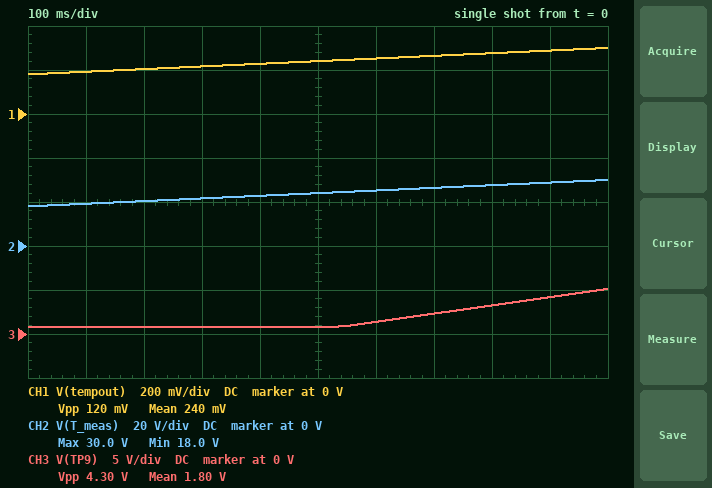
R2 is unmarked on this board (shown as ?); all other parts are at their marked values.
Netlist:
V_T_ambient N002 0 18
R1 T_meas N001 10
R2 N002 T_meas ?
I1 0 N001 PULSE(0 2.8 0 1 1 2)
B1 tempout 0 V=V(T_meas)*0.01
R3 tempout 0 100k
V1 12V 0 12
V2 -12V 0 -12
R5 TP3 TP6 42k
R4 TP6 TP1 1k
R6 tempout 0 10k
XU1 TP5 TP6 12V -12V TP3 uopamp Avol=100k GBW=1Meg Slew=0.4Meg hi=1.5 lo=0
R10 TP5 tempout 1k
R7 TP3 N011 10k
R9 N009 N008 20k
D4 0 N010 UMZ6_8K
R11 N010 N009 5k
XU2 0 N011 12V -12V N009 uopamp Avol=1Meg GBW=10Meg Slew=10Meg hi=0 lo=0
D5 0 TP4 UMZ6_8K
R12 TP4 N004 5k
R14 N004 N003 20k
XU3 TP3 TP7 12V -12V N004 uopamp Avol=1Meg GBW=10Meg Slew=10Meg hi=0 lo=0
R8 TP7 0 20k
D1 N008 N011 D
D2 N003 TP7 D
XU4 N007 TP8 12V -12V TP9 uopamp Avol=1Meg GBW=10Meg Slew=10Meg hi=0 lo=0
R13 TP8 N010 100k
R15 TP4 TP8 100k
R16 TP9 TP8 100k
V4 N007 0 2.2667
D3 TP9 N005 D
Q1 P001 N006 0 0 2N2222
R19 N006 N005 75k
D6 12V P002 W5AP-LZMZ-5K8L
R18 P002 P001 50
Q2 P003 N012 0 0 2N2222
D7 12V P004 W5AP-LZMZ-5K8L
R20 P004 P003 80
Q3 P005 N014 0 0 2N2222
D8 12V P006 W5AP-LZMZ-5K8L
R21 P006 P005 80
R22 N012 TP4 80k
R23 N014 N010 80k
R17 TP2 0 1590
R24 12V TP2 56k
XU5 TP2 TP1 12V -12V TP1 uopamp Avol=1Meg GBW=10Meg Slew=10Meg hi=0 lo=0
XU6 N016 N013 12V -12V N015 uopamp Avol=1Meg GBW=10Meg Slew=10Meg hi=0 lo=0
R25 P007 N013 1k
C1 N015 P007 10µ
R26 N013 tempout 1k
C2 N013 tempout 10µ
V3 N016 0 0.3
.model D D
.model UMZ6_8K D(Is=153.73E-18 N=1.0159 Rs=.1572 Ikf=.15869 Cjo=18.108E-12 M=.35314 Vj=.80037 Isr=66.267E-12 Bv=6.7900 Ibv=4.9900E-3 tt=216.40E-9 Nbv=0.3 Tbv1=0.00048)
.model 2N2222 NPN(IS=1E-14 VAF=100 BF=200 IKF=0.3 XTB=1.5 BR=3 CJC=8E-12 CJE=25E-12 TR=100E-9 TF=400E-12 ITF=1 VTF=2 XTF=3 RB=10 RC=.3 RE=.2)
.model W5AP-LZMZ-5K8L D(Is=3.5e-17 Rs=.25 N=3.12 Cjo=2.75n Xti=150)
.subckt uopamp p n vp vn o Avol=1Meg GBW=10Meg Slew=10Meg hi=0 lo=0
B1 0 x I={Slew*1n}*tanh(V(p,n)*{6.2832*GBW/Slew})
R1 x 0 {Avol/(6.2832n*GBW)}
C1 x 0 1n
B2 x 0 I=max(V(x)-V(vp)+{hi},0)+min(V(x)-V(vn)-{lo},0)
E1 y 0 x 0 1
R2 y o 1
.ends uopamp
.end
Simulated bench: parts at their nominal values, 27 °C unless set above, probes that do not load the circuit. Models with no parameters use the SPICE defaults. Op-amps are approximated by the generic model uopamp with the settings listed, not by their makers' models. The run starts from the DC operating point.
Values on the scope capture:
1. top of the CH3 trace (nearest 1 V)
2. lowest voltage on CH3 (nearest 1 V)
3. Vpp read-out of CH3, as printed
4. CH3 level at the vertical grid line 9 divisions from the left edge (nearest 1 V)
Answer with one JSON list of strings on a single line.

["5 V", "1 V", "4.30 V", "4 V"]
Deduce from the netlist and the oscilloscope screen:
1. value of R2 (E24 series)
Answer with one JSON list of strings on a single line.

["4.3 Ω"]
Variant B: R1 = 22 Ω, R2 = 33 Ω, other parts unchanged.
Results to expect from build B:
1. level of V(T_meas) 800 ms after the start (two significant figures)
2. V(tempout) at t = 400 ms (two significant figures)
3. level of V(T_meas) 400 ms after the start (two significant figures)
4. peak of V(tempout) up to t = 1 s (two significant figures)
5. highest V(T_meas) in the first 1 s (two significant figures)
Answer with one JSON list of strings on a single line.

["92 V", "550 mV", "55 V", "1.1 V", "110 V"]
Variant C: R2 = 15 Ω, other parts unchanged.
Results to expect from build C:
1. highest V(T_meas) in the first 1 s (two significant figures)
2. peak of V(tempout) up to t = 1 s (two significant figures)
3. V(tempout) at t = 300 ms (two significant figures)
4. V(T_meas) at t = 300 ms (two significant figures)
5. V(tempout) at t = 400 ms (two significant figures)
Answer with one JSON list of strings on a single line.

["60 V", "600 mV", "310 mV", "31 V", "350 mV"]
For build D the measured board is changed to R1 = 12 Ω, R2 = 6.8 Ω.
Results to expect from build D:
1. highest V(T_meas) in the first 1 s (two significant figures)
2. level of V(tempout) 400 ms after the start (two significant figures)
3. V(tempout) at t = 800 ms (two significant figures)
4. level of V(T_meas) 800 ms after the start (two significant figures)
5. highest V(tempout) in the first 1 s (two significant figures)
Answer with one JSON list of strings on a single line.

["37 V", "260 mV", "330 mV", "33 V", "370 mV"]
